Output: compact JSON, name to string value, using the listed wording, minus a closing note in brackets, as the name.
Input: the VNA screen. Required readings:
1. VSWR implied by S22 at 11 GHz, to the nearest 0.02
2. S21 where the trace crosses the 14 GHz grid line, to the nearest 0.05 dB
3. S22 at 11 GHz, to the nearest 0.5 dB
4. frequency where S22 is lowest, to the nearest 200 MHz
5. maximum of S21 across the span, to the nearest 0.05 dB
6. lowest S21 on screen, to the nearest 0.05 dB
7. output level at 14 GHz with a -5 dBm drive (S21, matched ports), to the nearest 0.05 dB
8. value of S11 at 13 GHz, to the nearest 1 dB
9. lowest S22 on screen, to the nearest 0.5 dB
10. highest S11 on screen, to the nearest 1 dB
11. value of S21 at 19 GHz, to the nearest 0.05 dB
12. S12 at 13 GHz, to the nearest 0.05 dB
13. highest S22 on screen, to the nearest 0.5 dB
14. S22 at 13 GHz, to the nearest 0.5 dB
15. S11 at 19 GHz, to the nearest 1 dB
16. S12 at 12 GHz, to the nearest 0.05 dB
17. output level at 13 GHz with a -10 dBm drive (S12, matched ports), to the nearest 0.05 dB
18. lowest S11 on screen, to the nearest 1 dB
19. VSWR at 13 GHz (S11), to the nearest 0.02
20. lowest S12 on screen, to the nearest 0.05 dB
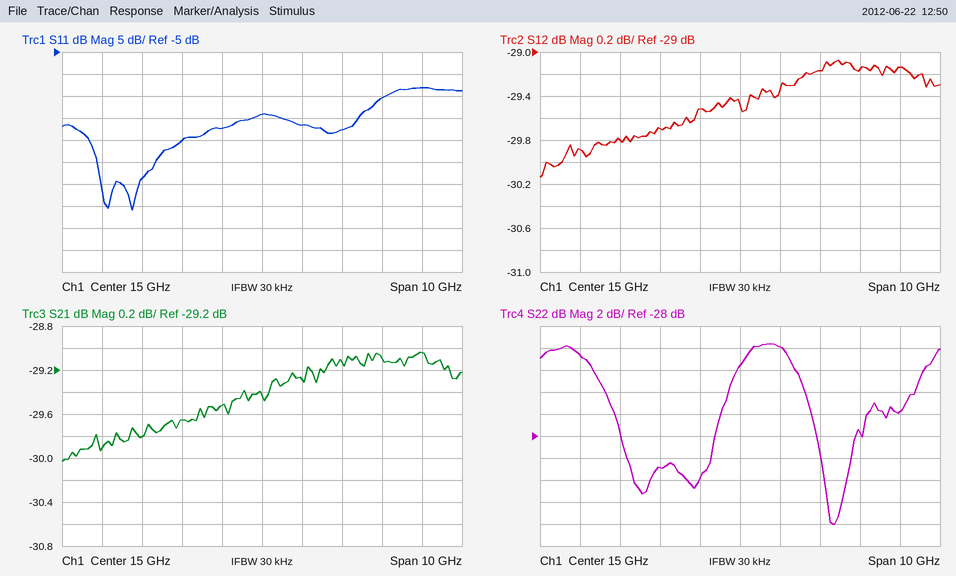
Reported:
{"VSWR implied by S22 at 11 GHz, to the nearest 0.02": "1.20", "S21 where the trace crosses the 14 GHz grid line, to the nearest 0.05 dB": "-29.50 dB", "S22 at 11 GHz, to the nearest 0.5 dB": "-20.5 dB", "frequency where S22 is lowest, to the nearest 200 MHz": "17.4 GHz", "maximum of S21 across the span, to the nearest 0.05 dB": "-29.05 dB", "lowest S21 on screen, to the nearest 0.05 dB": "-30.05 dB", "output level at 14 GHz with a -5 dBm drive (S21, matched ports), to the nearest 0.05 dB": "-34.50 dBm", "value of S11 at 13 GHz, to the nearest 1 dB": "-25 dB", "lowest S22 on screen, to the nearest 0.5 dB": "-36.0 dB", "highest S11 on screen, to the nearest 1 dB": "-13 dB", "value of S21 at 19 GHz, to the nearest 0.05 dB": "-29.05 dB", "S12 at 13 GHz, to the nearest 0.05 dB": "-29.70 dB", "highest S22 on screen, to the nearest 0.5 dB": "-19.5 dB", "S22 at 13 GHz, to the nearest 0.5 dB": "-31.0 dB", "S11 at 19 GHz, to the nearest 1 dB": "-13 dB", "S12 at 12 GHz, to the nearest 0.05 dB": "-29.80 dB", "output level at 13 GHz with a -10 dBm drive (S12, matched ports), to the nearest 0.05 dB": "-39.70 dBm", "lowest S11 on screen, to the nearest 1 dB": "-41 dB", "VSWR at 13 GHz (S11), to the nearest 0.02": "1.12", "lowest S12 on screen, to the nearest 0.05 dB": "-30.15 dB"}
